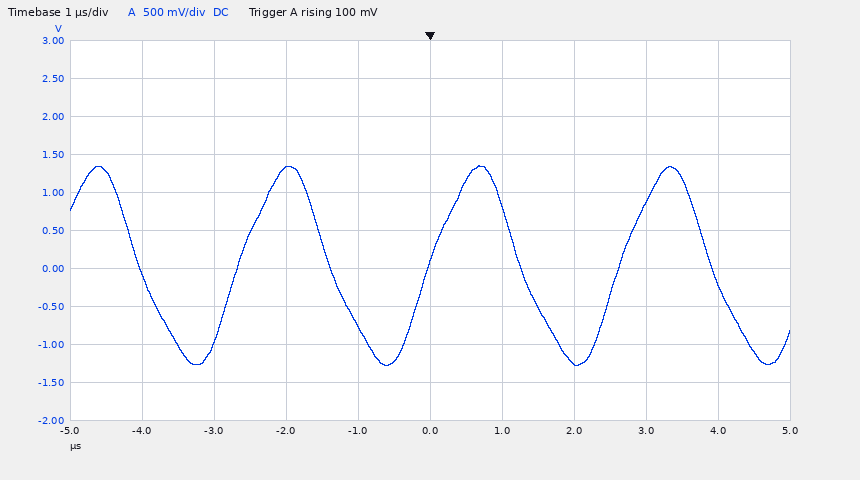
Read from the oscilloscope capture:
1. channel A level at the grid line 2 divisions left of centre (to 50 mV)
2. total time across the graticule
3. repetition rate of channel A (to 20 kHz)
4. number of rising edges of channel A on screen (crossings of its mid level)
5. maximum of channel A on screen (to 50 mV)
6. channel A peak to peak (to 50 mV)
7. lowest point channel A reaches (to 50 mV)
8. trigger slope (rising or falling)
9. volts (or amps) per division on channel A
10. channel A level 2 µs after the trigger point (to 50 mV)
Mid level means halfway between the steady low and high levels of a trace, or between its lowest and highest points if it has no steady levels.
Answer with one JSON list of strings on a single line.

["1.30 V", "10 µs", "380 kHz", "3", "1.35 V", "2.65 V", "-1.30 V", "rising", "500 mV", "-1.25 V"]
